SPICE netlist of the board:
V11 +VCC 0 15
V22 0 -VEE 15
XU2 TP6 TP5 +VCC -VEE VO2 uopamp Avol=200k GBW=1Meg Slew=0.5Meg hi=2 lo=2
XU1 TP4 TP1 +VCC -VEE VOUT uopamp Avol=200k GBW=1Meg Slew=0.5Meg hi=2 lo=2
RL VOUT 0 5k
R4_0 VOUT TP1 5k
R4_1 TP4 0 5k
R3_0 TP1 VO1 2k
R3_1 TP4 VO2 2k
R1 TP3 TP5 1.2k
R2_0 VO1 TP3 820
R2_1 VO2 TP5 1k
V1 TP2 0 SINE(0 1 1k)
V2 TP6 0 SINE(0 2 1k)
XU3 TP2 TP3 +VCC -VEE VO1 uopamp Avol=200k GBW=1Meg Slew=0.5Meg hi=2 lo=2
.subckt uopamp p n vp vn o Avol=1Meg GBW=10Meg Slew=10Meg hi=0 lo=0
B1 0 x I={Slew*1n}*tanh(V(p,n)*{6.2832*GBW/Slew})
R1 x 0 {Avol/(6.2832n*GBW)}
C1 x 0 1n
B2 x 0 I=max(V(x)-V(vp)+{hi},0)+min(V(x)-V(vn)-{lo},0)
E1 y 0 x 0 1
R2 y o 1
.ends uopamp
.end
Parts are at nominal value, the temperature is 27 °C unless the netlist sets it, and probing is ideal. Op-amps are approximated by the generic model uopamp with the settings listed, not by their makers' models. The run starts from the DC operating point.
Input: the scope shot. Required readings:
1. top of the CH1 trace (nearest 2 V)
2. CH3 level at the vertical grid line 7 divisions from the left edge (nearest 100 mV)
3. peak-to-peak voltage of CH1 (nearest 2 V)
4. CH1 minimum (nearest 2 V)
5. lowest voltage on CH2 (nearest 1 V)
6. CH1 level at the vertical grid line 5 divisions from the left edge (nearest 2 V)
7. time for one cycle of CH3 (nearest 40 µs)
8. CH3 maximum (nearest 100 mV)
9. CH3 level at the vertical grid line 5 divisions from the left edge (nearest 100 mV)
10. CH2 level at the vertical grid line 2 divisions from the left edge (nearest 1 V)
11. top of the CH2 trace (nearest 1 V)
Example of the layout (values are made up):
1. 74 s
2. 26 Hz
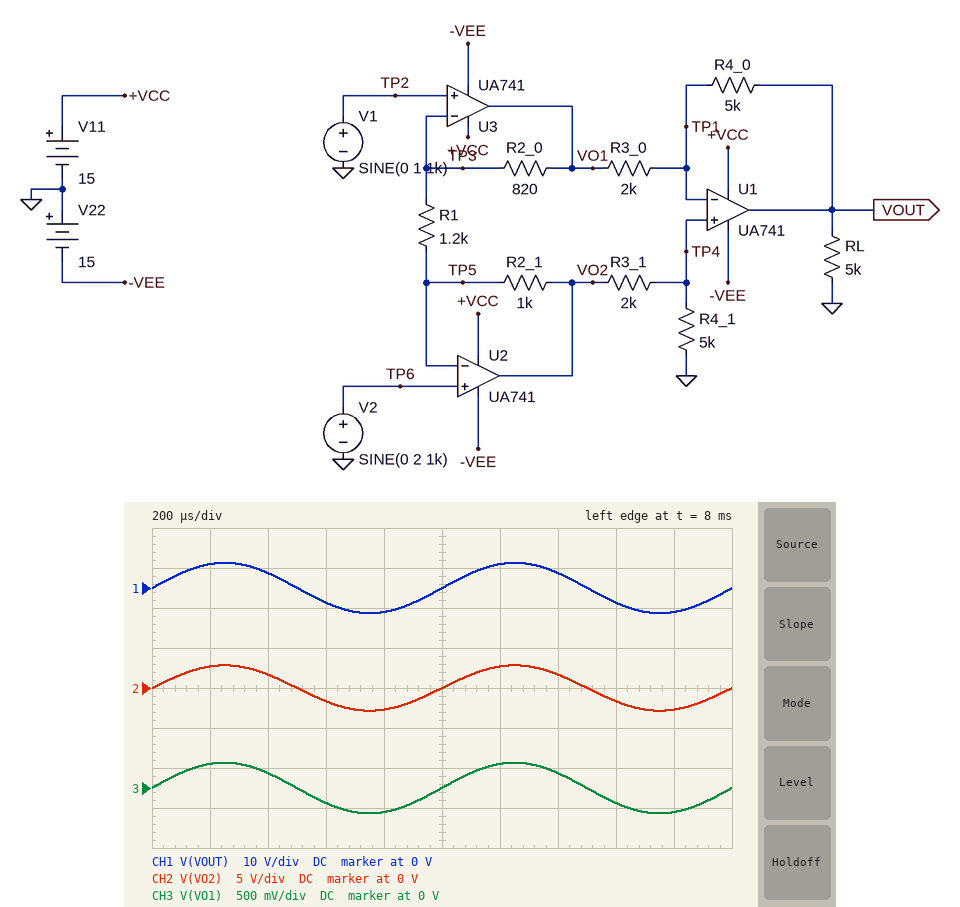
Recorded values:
1. 6 V
2. 200 mV
3. 12 V
4. -6 V
5. -3 V
6. 0 V
7. 1.00 ms
8. 300 mV
9. 0 V
10. 2 V
11. 3 V
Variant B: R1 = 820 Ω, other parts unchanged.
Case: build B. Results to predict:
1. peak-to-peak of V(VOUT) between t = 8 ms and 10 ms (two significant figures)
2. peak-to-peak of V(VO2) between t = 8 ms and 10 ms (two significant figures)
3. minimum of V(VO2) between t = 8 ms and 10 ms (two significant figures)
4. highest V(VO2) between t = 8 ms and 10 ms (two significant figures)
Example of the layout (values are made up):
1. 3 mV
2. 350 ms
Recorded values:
1. 16 V
2. 6.4 V
3. -3.2 V
4. 3.2 V
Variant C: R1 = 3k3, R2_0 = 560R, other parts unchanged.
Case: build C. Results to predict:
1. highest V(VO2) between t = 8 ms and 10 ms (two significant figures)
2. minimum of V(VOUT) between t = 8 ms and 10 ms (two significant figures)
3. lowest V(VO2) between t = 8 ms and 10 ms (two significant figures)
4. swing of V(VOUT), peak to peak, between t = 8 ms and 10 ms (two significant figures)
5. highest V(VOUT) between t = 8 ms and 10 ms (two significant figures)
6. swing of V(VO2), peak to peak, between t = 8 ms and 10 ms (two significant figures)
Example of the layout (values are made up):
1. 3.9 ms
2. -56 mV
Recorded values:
1. 2.3 V
2. -3.7 V
3. -2.3 V
4. 7.4 V
5. 3.7 V
6. 4.6 V
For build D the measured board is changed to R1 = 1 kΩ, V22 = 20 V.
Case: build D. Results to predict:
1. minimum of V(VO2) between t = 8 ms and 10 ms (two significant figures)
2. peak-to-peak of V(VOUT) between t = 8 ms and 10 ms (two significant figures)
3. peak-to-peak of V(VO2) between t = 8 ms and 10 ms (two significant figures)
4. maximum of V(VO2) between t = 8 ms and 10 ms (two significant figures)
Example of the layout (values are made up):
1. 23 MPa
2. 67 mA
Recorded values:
1. -3.0 V
2. 14 V
3. 6.0 V
4. 3.0 V
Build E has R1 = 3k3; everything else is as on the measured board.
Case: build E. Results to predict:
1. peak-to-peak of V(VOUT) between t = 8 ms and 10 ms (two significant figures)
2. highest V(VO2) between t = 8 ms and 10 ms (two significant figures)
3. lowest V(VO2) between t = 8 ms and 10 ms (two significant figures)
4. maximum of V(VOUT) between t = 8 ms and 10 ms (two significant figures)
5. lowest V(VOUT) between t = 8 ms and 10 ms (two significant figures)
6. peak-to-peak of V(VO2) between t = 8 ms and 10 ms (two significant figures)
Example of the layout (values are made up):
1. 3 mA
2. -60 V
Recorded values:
1. 7.8 V
2. 2.3 V
3. -2.3 V
4. 3.9 V
5. -3.9 V
6. 4.6 V
